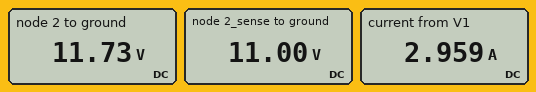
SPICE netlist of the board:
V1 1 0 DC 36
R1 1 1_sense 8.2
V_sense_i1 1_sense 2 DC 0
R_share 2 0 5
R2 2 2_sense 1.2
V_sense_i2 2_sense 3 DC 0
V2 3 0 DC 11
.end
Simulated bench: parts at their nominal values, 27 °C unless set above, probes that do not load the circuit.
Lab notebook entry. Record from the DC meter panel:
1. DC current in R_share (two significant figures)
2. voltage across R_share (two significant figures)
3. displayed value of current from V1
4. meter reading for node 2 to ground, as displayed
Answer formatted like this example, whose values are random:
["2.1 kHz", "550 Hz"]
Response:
["2.3 A", "12 V", "2.959 A", "11.73 V"]
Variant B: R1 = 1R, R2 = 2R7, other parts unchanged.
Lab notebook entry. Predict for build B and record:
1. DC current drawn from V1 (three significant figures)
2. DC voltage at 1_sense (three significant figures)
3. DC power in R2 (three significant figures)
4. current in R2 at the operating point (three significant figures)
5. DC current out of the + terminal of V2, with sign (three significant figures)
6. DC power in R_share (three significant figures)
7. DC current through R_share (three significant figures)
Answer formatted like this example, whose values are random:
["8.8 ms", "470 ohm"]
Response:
["10.5 A", "25.5 V", "78.1 W", "5.38 A", "-5.38 A", "130 W", "5.10 A"]
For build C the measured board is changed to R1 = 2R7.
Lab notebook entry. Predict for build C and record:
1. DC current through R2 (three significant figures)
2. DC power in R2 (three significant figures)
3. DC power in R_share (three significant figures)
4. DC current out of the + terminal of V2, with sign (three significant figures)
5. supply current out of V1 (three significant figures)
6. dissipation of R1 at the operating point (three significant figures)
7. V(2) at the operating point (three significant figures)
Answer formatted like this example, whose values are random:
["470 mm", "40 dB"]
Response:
["4.19 A", "21.1 W", "51.4 W", "-4.19 A", "7.40 A", "148 W", "16.0 V"]
